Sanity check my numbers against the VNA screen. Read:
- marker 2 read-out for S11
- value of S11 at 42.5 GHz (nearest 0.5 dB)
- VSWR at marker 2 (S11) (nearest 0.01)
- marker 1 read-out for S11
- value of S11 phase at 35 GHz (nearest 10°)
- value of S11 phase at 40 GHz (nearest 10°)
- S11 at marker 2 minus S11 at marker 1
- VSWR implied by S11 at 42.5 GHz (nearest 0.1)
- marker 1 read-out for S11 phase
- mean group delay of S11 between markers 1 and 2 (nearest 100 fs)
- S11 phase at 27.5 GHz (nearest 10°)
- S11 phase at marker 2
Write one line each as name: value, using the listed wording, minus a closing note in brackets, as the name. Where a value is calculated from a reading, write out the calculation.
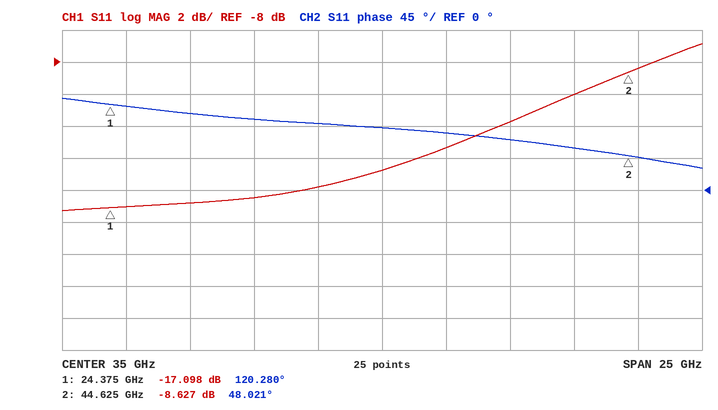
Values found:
marker 2 read-out for S11: -8.627 dB
value of S11 at 42.5 GHz: -10.0 dB
VSWR at marker 2 (S11): (1 + 0.3704)/(1 − 0.3704) ≈ 2.18
marker 1 read-out for S11: -17.098 dB
value of S11 phase at 35 GHz: 90°
value of S11 phase at 40 GHz: 70°
S11 at marker 2 minus S11 at marker 1: -8.627 − (-17.098) = 8.471 dB
VSWR implied by S11 at 42.5 GHz: |Γ| = 10^(-10/20) = 0.3162; VSWR = (1 + 0.3162)/(1 − 0.3162) ≈ 1.9
marker 1 read-out for S11 phase: 120.280°
mean group delay of S11 between markers 1 and 2: −(48.021° − (120.28°))/(360° × 20.25 GHz) ≈ 9.9 ps
S11 phase at 27.5 GHz: 110°
S11 phase at marker 2: 48.021°
